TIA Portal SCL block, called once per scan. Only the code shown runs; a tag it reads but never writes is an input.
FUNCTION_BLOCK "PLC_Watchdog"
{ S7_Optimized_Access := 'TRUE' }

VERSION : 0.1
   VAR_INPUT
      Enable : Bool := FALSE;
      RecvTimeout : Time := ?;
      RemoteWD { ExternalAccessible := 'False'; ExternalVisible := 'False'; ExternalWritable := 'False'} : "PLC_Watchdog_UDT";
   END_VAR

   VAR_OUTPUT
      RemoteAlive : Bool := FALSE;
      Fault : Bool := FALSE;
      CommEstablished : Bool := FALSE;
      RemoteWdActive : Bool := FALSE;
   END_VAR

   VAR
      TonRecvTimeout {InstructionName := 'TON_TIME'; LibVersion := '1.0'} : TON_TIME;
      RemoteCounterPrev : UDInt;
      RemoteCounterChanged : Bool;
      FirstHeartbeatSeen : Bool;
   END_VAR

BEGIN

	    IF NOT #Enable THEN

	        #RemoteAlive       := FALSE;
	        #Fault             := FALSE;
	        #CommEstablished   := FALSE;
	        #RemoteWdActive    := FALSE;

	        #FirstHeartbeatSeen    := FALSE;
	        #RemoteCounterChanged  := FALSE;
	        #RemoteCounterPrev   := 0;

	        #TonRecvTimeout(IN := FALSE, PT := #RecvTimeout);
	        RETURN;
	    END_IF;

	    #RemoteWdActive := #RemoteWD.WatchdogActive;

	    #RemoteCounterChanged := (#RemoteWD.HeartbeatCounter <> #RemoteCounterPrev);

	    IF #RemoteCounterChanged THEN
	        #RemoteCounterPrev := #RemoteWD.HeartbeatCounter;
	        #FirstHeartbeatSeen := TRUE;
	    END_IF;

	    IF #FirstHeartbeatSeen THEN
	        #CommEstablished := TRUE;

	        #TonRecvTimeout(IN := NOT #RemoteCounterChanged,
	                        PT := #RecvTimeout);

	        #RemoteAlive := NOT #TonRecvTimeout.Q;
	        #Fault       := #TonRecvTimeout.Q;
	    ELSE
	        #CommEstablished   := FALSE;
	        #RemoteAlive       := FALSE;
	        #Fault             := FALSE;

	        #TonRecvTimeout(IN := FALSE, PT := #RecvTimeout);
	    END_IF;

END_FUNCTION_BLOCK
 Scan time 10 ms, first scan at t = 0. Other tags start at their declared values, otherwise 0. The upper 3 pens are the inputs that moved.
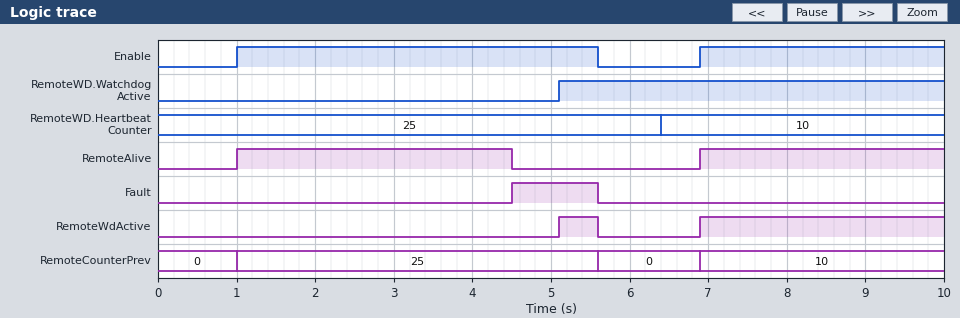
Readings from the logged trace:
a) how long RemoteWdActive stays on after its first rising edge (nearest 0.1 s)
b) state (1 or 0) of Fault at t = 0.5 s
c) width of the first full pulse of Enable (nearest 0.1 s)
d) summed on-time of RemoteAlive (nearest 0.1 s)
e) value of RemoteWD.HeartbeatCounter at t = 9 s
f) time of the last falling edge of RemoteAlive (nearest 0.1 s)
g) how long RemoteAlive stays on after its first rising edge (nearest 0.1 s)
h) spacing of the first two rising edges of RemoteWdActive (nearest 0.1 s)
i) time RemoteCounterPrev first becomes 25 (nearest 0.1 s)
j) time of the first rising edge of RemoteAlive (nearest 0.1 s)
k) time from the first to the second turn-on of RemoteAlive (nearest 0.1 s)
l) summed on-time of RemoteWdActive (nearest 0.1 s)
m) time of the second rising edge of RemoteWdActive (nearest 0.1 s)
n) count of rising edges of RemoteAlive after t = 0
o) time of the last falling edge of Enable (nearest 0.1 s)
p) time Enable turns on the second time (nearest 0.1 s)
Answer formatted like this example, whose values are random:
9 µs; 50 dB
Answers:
0.5 s; 0; 4.6 s; 6.6 s; 10; 4.5 s; 3.5 s; 1.8 s; 1.0 s; 1.0 s; 5.9 s; 3.6 s; 6.9 s; 2; 5.6 s; 6.9 s
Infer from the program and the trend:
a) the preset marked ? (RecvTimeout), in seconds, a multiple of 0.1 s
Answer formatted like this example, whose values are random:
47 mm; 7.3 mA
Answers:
3.5 s
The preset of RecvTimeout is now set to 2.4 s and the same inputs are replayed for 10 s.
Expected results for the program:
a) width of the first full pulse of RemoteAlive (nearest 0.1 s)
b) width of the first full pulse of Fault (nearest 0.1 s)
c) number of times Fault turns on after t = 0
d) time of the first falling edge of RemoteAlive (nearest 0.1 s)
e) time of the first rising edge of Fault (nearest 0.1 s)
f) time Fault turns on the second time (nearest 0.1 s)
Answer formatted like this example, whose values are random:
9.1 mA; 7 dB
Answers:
2.4 s; 2.2 s; 2; 3.4 s; 3.4 s; 9.3 s
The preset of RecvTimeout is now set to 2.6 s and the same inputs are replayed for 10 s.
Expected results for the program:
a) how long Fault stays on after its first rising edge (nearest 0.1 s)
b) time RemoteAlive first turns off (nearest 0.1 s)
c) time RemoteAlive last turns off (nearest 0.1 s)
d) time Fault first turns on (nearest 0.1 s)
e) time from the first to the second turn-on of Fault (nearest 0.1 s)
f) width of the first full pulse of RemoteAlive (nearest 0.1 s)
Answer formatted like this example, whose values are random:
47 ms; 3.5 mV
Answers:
2.0 s; 3.6 s; 9.5 s; 3.6 s; 5.9 s; 2.6 s
